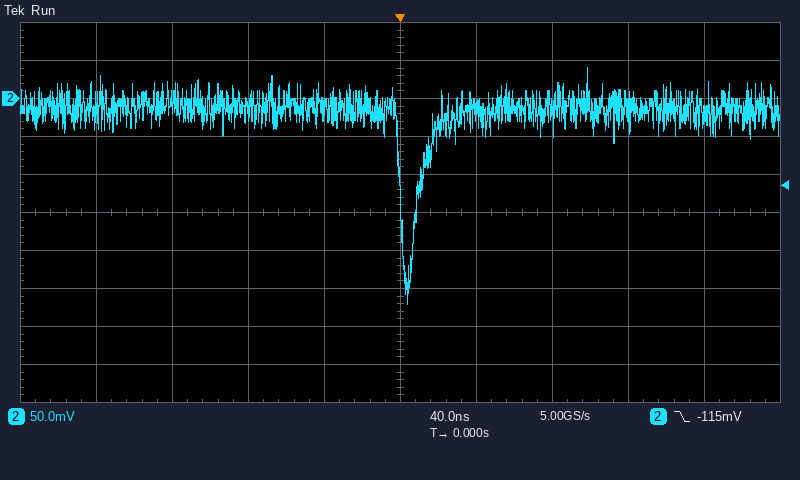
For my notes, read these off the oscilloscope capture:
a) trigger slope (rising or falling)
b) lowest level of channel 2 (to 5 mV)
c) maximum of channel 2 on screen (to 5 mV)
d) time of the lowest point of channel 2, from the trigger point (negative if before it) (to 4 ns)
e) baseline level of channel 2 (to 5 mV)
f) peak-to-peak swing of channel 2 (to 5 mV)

falling
-270 mV
40 mV
+4 ns
-15 mV
310 mV
